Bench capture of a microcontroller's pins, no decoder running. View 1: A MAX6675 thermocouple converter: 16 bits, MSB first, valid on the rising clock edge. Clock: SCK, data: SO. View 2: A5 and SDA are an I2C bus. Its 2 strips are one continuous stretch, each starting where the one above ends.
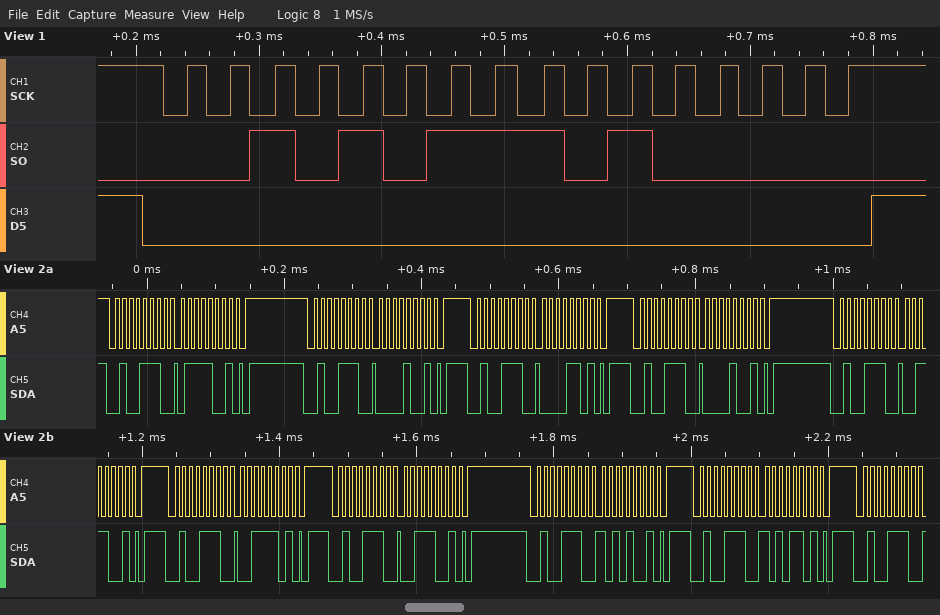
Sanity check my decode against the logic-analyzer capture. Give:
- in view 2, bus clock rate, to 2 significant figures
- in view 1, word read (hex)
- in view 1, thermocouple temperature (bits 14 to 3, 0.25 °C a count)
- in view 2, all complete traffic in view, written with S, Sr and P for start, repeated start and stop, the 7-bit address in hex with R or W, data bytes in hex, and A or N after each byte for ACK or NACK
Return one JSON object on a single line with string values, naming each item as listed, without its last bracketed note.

{"in view 2, bus clock rate, to 2 significant figures": "100 kHz", "in view 1, word read": "0x2BA0", "in view 1, thermocouple temperature": "349.00 °C", "in view 2, all complete traffic in view, written with S, Sr and P for start, repeated start and stop, the 7-bit address in hex with R or W, data bytes in hex, and A or N after each byte for ACK or NACK": "S 27W A 79 A P S 27W A 09 A P S 27W A 0D A P S 27W A 09 A P S 27W A 39 A P S 27W A 3D A P S 27W A 39 A P S 27W A A9 A P S 27W A AD A P S 27W A"}
